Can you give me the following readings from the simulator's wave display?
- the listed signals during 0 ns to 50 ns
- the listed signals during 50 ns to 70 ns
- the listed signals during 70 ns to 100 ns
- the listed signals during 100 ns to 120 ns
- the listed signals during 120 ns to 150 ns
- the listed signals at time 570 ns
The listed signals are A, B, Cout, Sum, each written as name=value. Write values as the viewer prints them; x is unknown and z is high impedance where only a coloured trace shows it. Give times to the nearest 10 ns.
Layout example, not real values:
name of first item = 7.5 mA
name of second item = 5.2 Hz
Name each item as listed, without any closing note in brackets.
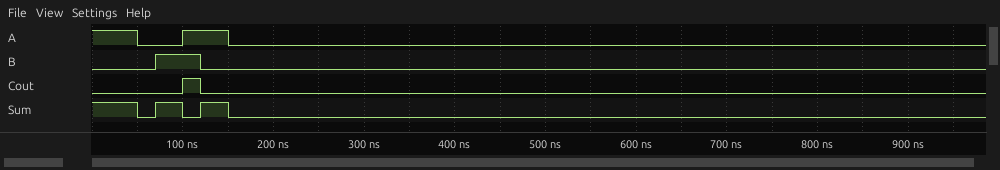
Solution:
the listed signals during 0 ns to 50 ns = A=1, B=0, Cout=0, Sum=1
the listed signals during 50 ns to 70 ns = A=0, B=0, Cout=0, Sum=0
the listed signals during 70 ns to 100 ns = A=0, B=1, Cout=0, Sum=1
the listed signals during 100 ns to 120 ns = A=1, B=1, Cout=1, Sum=0
the listed signals during 120 ns to 150 ns = A=1, B=0, Cout=0, Sum=1
the listed signals at time 570 ns = A=0, B=0, Cout=0, Sum=0
